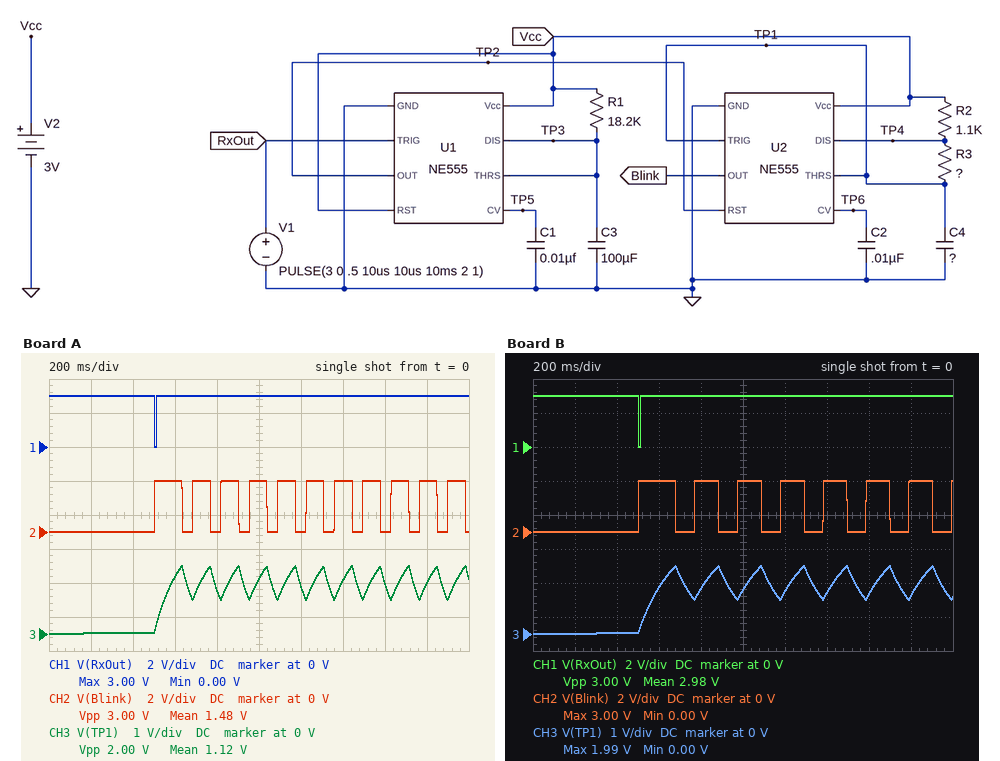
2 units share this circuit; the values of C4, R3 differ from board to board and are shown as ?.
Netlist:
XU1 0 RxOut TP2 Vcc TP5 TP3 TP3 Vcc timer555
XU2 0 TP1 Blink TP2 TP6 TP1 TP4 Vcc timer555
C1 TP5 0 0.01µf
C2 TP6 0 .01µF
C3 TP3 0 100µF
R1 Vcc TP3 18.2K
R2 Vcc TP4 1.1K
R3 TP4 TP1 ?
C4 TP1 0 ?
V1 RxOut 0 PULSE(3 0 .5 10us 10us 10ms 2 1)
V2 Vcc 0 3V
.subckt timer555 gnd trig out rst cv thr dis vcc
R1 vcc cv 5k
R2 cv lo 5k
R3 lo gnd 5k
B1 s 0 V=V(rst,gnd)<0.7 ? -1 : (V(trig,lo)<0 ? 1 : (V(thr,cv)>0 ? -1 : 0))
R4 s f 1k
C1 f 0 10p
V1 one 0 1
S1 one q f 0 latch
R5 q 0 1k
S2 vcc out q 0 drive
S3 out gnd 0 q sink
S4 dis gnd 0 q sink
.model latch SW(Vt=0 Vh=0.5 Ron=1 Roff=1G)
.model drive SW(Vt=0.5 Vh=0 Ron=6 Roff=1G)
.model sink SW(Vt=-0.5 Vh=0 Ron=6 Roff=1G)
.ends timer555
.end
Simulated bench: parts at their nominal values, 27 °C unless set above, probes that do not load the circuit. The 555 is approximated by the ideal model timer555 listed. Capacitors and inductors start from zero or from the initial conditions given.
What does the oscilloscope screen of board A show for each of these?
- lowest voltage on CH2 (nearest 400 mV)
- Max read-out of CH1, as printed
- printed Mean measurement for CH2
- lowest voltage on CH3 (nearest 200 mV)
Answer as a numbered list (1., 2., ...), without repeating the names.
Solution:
1. 0 V
2. 3.00 V
3. 1.48 V
4. 0 V
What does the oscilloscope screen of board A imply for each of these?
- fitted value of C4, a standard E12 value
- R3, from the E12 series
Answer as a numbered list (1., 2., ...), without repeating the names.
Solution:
1. 47 µF
2. 1.5 kΩ
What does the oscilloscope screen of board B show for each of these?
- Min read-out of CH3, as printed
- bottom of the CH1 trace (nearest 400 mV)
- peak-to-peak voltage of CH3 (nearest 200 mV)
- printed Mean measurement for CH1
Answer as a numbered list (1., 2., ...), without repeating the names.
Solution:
1. 0.00 V
2. 0 V
3. 2.0 V
4. 2.98 V
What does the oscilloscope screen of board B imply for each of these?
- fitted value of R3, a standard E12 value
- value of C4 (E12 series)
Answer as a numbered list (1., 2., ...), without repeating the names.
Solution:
1. 3.9 kΩ
2. 33 µF
